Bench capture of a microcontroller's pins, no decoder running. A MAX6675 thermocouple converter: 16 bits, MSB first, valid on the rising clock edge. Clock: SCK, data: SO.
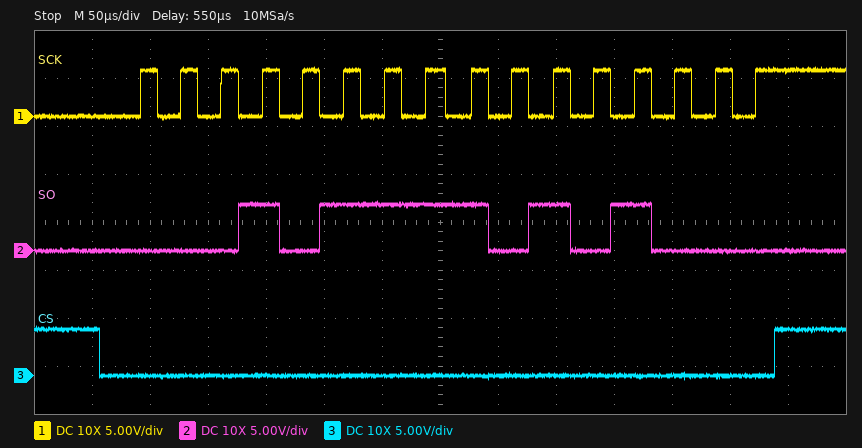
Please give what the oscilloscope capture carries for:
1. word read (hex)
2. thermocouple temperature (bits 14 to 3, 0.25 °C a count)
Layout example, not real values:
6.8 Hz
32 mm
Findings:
0x17A8
189.25 °C
